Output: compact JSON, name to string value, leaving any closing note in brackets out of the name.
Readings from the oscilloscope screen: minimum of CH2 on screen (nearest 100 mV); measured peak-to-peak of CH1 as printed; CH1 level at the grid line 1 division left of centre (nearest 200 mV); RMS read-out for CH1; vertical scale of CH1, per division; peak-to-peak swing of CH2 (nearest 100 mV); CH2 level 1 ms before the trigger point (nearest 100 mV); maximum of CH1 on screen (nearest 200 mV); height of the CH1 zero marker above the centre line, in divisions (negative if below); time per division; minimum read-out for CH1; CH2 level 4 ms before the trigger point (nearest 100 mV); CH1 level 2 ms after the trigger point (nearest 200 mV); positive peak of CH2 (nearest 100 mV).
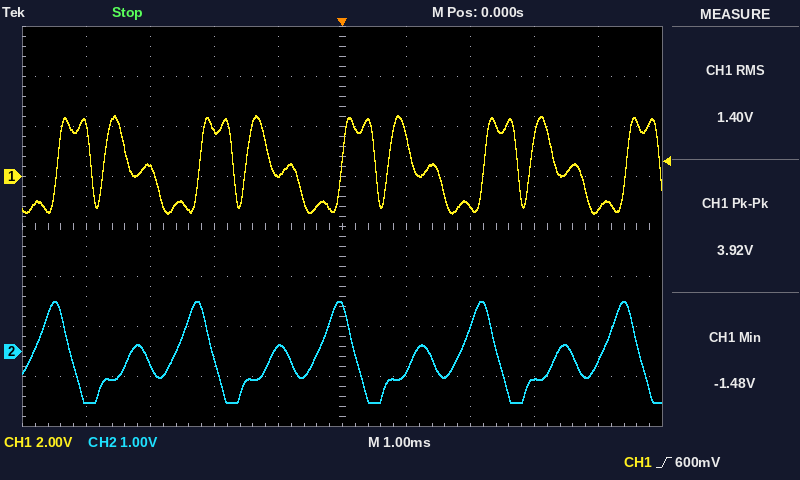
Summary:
{"minimum of CH2 on screen": "-1.0 V", "measured peak-to-peak of CH1 as printed": "3.92 V", "CH1 level at the grid line 1 division left of centre": "0.0 V", "RMS read-out for CH1": "1.40 V", "vertical scale of CH1, per division": "2 V", "peak-to-peak swing of CH2": "2.0 V", "CH2 level 1 ms before the trigger point": "100 mV", "maximum of CH1 on screen": "2.4 V", "height of the CH1 zero marker above the centre line, in divisions": "+1.0 div", "time per division": "1 ms", "minimum read-out for CH1": "-1.48 V", "CH2 level 4 ms before the trigger point": "-1.0 V", "CH1 level 2 ms after the trigger point": "-1.2 V", "positive peak of CH2": "1.0 V"}
